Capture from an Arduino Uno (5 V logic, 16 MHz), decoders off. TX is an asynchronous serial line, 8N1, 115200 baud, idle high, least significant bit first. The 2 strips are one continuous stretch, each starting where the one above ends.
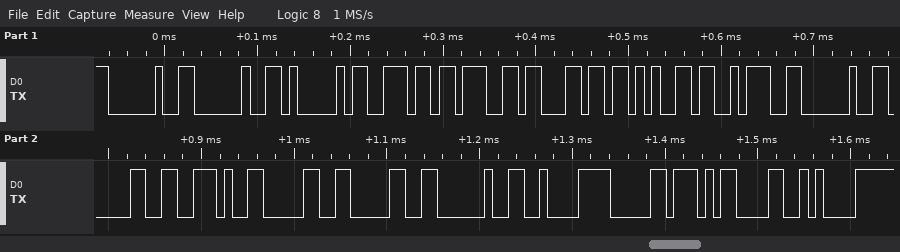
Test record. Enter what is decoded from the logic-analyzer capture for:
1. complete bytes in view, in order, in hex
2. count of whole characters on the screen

0x20 0x20 0x41 0x6E 0x67 0x6C 0x65 0x3A 0x20 0x30 0x2E 0x30 0x30 0x20 0xC2 0xB0 0x0D 0x0A
18
